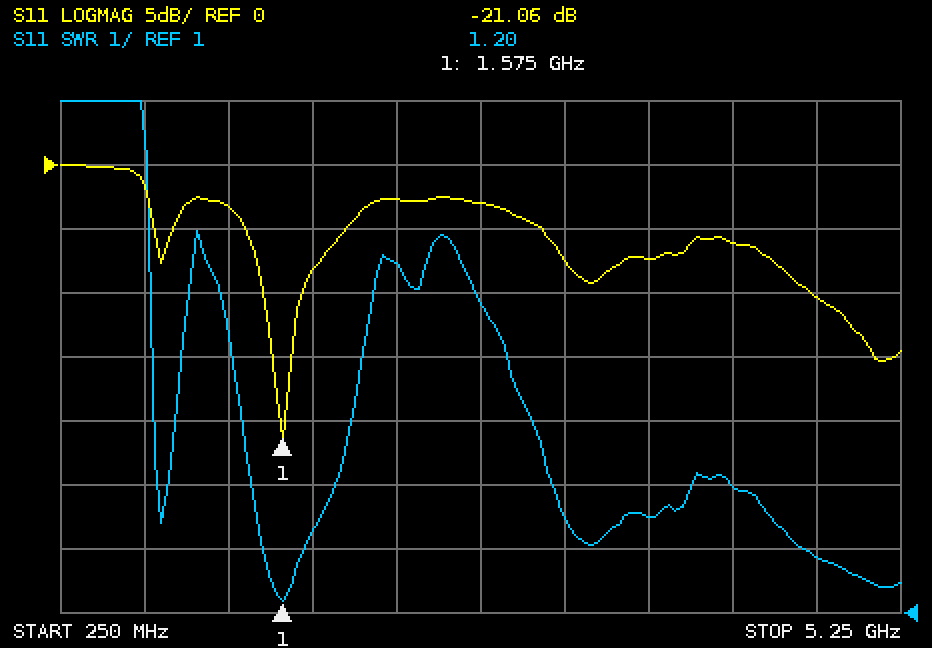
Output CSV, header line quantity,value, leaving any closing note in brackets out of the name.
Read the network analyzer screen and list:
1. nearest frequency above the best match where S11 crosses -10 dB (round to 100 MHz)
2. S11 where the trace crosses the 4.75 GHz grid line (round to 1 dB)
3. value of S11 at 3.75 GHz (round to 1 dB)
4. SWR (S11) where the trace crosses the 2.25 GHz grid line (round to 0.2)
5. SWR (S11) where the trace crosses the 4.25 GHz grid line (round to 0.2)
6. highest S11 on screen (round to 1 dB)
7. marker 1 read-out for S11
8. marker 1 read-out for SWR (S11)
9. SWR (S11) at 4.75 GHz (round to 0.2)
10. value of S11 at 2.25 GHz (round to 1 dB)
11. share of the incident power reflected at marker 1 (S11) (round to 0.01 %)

quantity,value
nearest frequency above the best match where S11 crosses -10 dB,1.7 GHz
S11 where the trace crosses the 4.75 GHz grid line,-10 dB
value of S11 at 3.75 GHz,-7 dB
SWR (S11) where the trace crosses the 2.25 GHz grid line,6.4
SWR (S11) where the trace crosses the 4.25 GHz grid line,3.0
highest S11 on screen,0 dB
marker 1 read-out for S11,-21.06 dB
marker 1 read-out for SWR,1.20
SWR (S11) at 4.75 GHz,1.8
value of S11 at 2.25 GHz,-3 dB
share of the incident power reflected at marker 1 (S11),0.78 %
